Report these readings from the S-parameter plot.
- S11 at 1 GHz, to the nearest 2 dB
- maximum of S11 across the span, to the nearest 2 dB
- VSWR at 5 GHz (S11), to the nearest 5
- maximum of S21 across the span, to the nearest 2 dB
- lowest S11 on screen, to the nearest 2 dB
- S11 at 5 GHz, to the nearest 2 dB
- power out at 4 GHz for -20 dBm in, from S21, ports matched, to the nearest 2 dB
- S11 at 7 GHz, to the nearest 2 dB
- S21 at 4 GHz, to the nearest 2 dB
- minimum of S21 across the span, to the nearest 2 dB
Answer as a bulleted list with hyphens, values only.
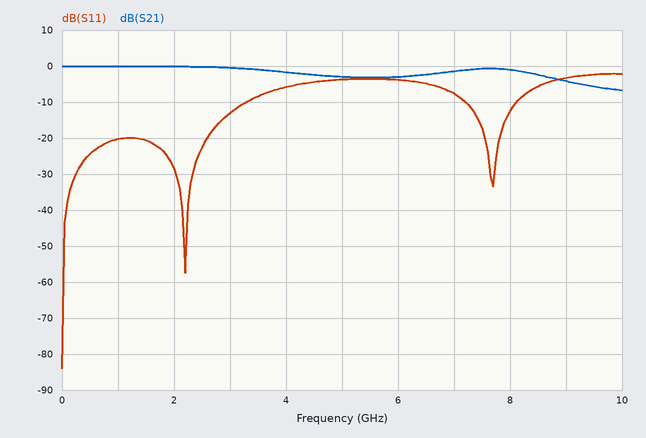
- -20 dB
- -2 dB
- 5
- 0 dB
- -84 dB
- -4 dB
- -22 dBm
- -8 dB
- -2 dB
- -6 dB
